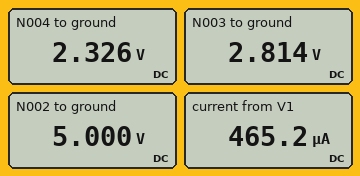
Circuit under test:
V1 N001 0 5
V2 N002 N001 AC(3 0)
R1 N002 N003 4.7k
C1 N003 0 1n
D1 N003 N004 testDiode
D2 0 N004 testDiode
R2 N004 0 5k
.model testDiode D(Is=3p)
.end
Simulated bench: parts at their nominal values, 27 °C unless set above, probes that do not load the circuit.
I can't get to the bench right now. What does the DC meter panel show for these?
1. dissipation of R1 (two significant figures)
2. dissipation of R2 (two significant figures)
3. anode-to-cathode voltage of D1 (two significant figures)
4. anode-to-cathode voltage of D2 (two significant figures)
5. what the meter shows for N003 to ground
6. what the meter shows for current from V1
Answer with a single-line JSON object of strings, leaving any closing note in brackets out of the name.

{"dissipation of R1": "1.0 mW", "dissipation of R2": "1.1 mW", "anode-to-cathode voltage of D1": "490 mV", "anode-to-cathode voltage of D2": "-2.3 V", "what the meter shows for N003 to ground": "2.814 V", "what the meter shows for current from V1": "465.2 µA"}
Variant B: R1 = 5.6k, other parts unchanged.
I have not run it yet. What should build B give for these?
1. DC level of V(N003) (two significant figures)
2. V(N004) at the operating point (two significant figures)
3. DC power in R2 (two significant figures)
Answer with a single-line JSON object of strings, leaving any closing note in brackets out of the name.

{"DC level of V(N003)": "2.6 V", "V(N004) at the operating point": "2.1 V", "DC power in R2": "910 µW"}
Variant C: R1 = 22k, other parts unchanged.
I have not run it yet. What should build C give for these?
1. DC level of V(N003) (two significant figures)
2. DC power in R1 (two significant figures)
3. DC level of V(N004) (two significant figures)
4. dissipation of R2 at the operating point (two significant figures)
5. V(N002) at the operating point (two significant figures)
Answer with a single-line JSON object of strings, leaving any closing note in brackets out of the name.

{"DC level of V(N003)": "1.3 V", "DC power in R1": "620 µW", "DC level of V(N004)": "840 mV", "dissipation of R2 at the operating point": "140 µW", "V(N002) at the operating point": "5.0 V"}
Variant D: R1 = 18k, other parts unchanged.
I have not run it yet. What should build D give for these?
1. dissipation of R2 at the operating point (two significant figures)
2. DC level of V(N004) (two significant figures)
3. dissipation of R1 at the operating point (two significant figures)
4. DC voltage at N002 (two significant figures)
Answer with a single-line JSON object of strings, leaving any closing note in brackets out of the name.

{"dissipation of R2 at the operating point": "190 µW", "DC level of V(N004)": "990 mV", "dissipation of R1 at the operating point": "700 µW", "DC voltage at N002": "5.0 V"}
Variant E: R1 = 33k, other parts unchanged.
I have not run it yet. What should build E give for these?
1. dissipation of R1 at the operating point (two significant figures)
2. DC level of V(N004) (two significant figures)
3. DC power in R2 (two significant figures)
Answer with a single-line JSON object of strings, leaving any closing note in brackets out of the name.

{"dissipation of R1 at the operating point": "470 µW", "DC level of V(N004)": "600 mV", "DC power in R2": "72 µW"}
